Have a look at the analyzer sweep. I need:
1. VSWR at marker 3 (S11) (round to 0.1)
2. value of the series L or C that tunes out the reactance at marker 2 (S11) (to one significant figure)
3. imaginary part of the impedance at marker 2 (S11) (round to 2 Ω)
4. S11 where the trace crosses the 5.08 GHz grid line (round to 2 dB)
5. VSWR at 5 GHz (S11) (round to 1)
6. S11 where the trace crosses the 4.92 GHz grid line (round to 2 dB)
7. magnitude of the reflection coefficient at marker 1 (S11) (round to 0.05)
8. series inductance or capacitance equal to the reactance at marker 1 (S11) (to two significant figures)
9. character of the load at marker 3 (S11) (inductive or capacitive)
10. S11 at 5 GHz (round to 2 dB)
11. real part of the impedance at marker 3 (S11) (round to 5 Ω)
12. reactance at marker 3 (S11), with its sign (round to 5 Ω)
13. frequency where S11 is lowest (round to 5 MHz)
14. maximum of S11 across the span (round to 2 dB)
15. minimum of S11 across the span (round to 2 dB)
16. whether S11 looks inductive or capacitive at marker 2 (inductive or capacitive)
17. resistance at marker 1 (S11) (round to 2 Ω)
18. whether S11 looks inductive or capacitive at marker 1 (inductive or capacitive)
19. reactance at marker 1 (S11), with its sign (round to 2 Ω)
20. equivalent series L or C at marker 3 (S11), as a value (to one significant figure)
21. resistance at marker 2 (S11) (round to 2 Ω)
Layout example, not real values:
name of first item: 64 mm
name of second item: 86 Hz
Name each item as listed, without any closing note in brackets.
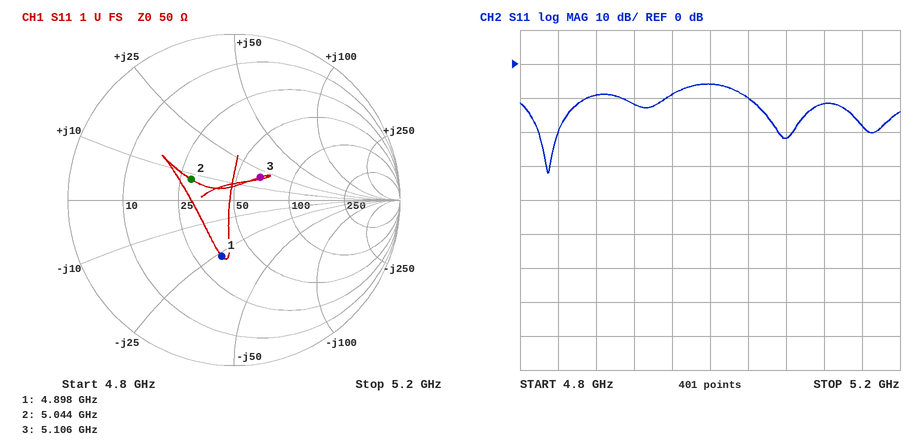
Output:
VSWR at marker 3 (S11): 1.5
value of the series L or C that tunes out the reactance at marker 2 (S11): 4 pF
imaginary part of the impedance at marker 2 (S11): +8 Ω
S11 where the trace crosses the 5.08 GHz grid line: -22 dB
VSWR at 5 GHz (S11): 3
S11 where the trace crosses the 4.92 GHz grid line: -12 dB
magnitude of the reflection coefficient at marker 1 (S11): 0.35
series inductance or capacitance equal to the reactance at marker 1 (S11): 1.2 pF
character of the load at marker 3 (S11): inductive
S11 at 5 GHz: -6 dB
real part of the impedance at marker 3 (S11): 65 Ω
reactance at marker 3 (S11), with its sign: +20 Ω
frequency where S11 is lowest: 4.830 GHz
maximum of S11 across the span: -6 dB
minimum of S11 across the span: -32 dB
whether S11 looks inductive or capacitive at marker 2: inductive
resistance at marker 1 (S11): 34 Ω
whether S11 looks inductive or capacitive at marker 1: capacitive
reactance at marker 1 (S11), with its sign: -26 Ω
equivalent series L or C at marker 3 (S11), as a value: 600 pH
resistance at marker 2 (S11): 28 Ω
